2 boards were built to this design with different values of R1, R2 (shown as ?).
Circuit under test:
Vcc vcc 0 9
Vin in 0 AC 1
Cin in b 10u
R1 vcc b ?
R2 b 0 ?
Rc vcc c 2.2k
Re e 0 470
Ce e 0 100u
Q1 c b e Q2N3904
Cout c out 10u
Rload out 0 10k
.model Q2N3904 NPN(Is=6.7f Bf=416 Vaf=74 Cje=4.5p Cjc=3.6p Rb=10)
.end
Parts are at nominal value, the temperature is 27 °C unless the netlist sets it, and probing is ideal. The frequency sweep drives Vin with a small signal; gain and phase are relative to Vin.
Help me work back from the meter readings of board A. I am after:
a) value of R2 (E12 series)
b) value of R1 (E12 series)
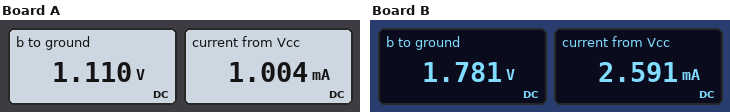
22 kΩ
150 kΩ
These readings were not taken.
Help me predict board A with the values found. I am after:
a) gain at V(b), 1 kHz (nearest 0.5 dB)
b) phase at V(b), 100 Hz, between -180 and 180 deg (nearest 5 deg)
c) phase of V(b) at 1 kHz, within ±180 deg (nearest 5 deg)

0 dB
0 deg
0 deg
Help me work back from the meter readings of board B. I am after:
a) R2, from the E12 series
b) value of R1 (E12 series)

6.8 kΩ
27 kΩ
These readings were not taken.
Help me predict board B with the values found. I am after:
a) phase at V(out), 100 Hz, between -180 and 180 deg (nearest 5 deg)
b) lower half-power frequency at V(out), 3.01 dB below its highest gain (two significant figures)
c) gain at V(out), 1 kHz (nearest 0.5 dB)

-125 deg
140 Hz
43.5 dB
